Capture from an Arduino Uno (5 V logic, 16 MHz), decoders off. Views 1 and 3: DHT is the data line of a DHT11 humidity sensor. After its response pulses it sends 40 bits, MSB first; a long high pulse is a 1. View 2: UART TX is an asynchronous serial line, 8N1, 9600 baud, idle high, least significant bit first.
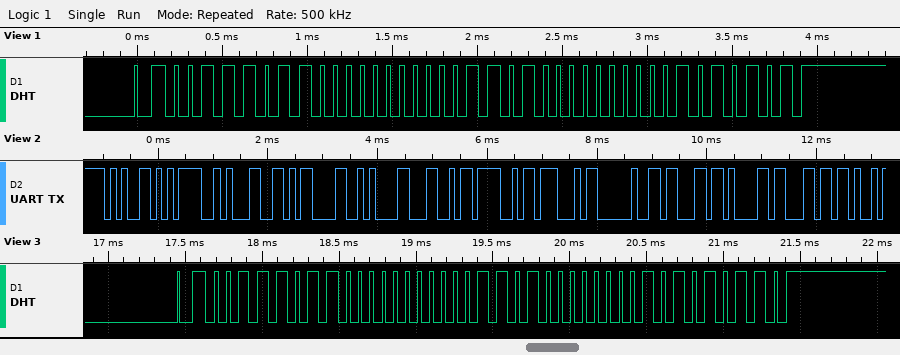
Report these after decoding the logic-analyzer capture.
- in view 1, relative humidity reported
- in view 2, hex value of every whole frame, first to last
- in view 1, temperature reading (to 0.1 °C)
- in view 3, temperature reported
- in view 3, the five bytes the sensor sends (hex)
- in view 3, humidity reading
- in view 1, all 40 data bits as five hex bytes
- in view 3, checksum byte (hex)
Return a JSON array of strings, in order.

["59 %", "0x65 0x3D 0x31 0x0D 0x0A 0x4C 0x4F 0x47 0x20 0x63 0x61 0x6C", "26.0 °C", "26.1 °C", "3B 00 1A 01 56", "59 %", "3B 00 1A 00 55", "0x56"]
